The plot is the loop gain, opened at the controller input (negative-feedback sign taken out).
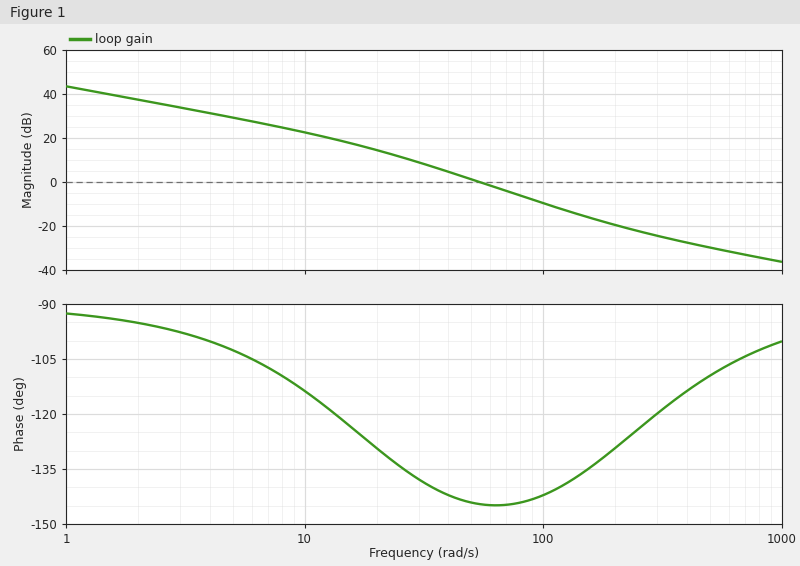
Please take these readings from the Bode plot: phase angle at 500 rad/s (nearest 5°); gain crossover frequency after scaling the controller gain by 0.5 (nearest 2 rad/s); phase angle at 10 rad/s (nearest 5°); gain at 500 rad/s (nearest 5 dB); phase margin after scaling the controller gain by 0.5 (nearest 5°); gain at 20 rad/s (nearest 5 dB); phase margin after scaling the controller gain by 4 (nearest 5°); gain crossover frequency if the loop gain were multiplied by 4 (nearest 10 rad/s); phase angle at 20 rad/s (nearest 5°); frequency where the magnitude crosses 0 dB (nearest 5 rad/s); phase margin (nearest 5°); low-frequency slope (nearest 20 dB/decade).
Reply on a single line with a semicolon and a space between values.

-110°; 36 rad/s; -115°; -30 dB; 40°; 15 dB; 40°; 120 rad/s; -130°; 55 rad/s; 35°; -20 dB/decade
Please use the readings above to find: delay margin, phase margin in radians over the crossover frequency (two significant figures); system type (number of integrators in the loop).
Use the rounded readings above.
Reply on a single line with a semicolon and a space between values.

0.011 s; 1
